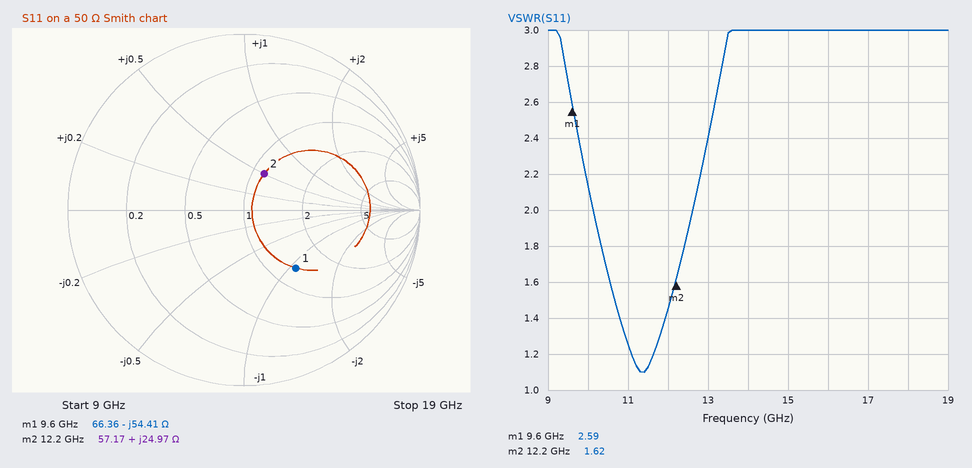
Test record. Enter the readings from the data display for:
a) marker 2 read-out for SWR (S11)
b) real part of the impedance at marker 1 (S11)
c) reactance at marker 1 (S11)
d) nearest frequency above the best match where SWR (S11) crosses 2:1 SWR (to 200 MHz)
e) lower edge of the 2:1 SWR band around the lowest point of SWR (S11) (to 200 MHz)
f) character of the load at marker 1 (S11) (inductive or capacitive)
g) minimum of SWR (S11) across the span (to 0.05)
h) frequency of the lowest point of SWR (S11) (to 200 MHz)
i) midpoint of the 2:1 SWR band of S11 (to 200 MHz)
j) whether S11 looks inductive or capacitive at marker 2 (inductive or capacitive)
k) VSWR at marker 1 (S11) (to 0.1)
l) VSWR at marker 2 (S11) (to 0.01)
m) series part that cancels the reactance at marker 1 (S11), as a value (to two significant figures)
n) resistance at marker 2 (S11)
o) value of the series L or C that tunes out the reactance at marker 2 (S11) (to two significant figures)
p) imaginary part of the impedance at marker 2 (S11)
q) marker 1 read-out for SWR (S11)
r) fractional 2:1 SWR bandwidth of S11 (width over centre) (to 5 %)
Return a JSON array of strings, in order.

["1.62", "66.36 Ω", "-54.41 Ω", "12.6 GHz", "10.2 GHz", "capacitive", "1.10", "11.4 GHz", "11.4 GHz", "inductive", "2.6", "1.62", "900 pH", "57.17 Ω", "520 fF", "+24.97 Ω", "2.59", "20 %"]
